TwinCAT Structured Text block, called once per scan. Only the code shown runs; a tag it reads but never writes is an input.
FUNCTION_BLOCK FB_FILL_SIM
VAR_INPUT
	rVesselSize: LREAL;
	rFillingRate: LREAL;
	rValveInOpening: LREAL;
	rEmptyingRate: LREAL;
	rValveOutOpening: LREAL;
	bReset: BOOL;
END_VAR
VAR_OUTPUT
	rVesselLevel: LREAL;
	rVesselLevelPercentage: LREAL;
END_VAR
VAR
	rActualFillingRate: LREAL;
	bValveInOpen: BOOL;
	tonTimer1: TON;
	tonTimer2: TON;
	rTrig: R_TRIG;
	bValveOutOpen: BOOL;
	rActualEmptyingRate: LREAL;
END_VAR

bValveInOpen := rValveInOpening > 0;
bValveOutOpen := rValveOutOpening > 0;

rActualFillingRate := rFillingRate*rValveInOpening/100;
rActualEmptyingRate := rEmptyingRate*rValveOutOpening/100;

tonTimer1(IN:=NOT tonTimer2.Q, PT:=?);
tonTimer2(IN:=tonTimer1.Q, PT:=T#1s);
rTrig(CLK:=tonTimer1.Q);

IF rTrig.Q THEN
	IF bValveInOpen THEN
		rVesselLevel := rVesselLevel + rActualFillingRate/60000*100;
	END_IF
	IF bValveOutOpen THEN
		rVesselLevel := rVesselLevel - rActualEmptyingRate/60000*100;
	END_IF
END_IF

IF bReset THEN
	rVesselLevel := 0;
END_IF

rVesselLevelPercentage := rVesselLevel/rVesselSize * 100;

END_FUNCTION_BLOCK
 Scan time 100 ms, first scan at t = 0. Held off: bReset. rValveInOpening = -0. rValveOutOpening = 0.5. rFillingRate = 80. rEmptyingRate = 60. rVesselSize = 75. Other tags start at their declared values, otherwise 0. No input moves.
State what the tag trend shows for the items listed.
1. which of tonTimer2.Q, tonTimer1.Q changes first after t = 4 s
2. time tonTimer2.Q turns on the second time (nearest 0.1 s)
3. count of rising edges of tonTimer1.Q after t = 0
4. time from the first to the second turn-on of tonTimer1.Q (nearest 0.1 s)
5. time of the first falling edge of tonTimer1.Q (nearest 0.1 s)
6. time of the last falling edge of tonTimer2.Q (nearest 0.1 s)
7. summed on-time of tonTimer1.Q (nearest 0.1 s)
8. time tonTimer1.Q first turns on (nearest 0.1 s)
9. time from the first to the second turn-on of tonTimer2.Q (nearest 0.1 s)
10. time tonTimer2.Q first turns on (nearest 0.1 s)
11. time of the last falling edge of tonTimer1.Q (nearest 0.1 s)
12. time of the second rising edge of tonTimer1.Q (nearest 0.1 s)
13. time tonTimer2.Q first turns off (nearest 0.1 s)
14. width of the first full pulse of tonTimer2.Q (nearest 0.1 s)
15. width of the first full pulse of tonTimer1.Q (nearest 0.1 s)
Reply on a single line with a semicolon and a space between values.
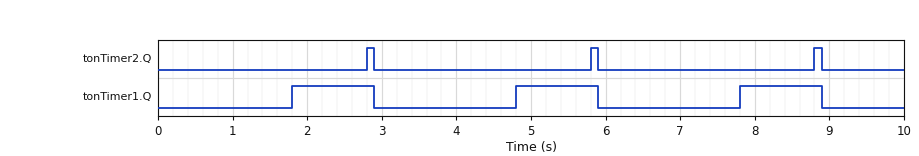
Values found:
tonTimer1.Q; 5.8 s; 3; 3.0 s; 2.9 s; 8.9 s; 3.3 s; 1.8 s; 3.0 s; 2.8 s; 8.9 s; 4.8 s; 2.9 s; 0.1 s; 1.1 s
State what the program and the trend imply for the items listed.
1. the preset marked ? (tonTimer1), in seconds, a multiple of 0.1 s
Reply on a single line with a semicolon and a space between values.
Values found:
1.8 s
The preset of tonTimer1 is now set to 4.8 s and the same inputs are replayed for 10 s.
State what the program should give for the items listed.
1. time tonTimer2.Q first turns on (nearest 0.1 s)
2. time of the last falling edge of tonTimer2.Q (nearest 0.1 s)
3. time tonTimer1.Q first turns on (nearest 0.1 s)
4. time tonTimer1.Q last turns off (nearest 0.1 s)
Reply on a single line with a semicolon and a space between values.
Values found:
5.8 s; 5.9 s; 4.8 s; 5.9 s
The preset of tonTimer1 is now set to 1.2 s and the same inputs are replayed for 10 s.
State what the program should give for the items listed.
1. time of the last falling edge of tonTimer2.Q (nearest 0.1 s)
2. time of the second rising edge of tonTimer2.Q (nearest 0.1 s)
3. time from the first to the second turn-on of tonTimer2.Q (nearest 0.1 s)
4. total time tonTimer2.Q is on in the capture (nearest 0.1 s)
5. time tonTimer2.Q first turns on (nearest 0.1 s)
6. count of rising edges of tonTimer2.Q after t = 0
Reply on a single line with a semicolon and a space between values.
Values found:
9.5 s; 4.6 s; 2.4 s; 0.4 s; 2.2 s; 4
